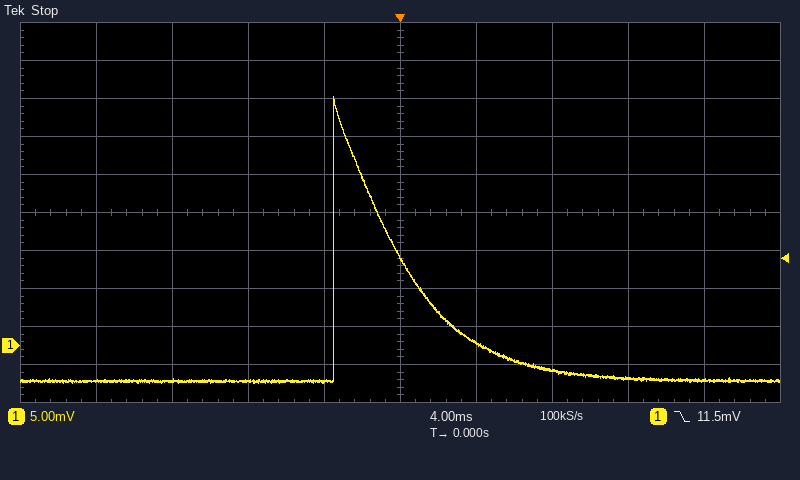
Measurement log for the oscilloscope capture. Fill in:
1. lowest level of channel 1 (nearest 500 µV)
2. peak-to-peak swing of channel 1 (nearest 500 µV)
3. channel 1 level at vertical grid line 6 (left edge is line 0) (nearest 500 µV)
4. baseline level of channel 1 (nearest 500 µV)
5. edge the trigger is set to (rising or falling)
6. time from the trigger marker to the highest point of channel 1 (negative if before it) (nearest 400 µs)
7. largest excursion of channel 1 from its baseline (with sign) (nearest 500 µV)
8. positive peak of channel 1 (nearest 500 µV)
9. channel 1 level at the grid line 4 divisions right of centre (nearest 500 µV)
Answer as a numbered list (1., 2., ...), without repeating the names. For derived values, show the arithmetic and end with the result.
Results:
1. -5.0 mV
2. 33.0 mV − (-5.0 mV) = 38.0 mV
3. 500 µV
4. -4.5 mV
5. falling
6. -3.6 ms
7. 33.0 mV − (-4.5 mV) = +37.5 mV
8. 33.0 mV
9. -4.5 mV
